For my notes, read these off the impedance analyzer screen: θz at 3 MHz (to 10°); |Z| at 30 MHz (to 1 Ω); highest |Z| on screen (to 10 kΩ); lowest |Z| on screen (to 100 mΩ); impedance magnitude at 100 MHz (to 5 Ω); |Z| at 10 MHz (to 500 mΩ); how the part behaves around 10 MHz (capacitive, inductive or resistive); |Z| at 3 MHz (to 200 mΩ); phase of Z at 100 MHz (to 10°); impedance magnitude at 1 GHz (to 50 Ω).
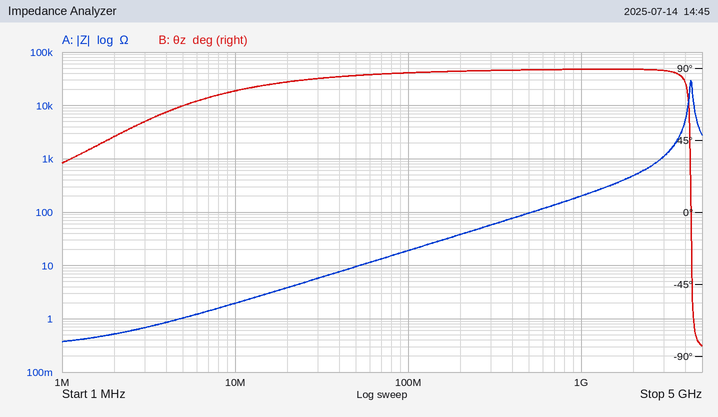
60°
6 Ω
30 kΩ
400 mΩ
20 Ω
2.0 Ω
inductive
600 mΩ
90°
200 Ω
